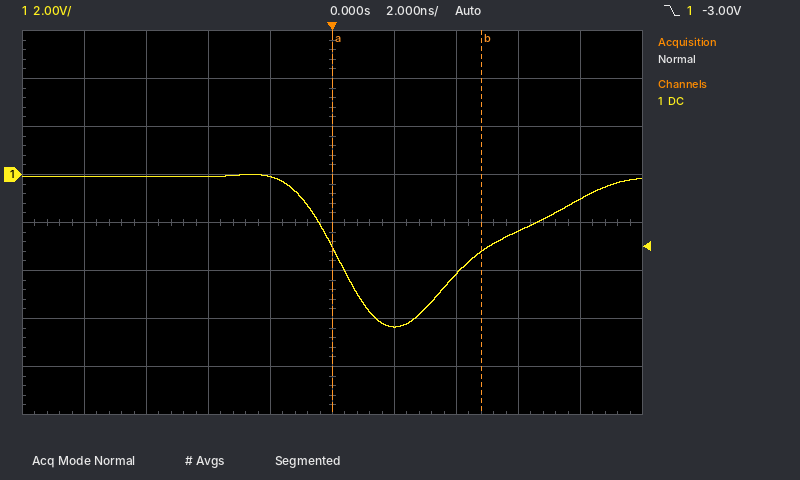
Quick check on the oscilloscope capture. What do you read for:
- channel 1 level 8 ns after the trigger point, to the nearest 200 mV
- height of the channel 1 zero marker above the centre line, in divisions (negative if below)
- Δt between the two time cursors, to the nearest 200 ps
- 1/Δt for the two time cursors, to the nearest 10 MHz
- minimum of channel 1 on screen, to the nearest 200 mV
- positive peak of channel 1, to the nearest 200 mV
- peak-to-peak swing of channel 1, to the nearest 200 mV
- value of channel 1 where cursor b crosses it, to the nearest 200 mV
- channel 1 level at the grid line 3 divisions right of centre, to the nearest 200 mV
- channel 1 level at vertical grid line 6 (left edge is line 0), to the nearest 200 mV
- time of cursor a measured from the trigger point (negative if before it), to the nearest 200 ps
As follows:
-1.0 V
+1.0 div
4.8 ns
210 MHz
-6.4 V
0.0 V
6.4 V
-3.2 V
-2.4 V
-6.4 V
0.0 ns
